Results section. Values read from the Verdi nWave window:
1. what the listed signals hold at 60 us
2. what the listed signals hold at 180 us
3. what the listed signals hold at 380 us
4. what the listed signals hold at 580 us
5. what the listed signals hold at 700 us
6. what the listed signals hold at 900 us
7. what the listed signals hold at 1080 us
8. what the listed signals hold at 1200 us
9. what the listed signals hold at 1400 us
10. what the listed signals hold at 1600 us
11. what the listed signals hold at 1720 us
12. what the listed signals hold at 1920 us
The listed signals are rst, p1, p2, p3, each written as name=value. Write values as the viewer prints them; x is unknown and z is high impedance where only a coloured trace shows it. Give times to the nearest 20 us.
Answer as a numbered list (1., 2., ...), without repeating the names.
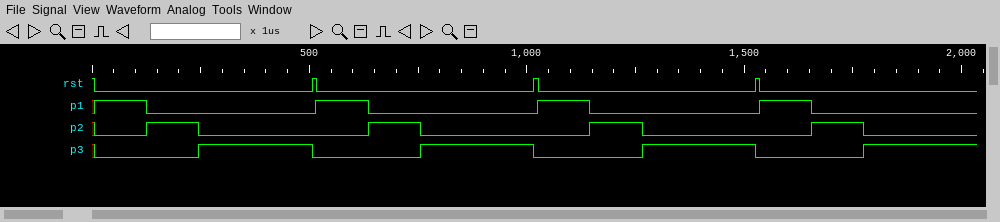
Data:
1. rst=0, p1=1, p2=0, p3=0
2. rst=0, p1=0, p2=1, p3=0
3. rst=0, p1=0, p2=0, p3=1
4. rst=0, p1=1, p2=0, p3=0
5. rst=0, p1=0, p2=1, p3=0
6. rst=0, p1=0, p2=0, p3=1
7. rst=0, p1=1, p2=0, p3=0
8. rst=0, p1=0, p2=1, p3=0
9. rst=0, p1=0, p2=0, p3=1
10. rst=0, p1=1, p2=0, p3=0
11. rst=0, p1=0, p2=1, p3=0
12. rst=0, p1=0, p2=0, p3=1
